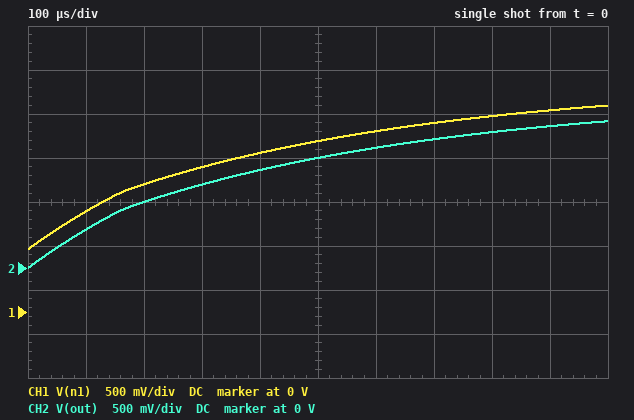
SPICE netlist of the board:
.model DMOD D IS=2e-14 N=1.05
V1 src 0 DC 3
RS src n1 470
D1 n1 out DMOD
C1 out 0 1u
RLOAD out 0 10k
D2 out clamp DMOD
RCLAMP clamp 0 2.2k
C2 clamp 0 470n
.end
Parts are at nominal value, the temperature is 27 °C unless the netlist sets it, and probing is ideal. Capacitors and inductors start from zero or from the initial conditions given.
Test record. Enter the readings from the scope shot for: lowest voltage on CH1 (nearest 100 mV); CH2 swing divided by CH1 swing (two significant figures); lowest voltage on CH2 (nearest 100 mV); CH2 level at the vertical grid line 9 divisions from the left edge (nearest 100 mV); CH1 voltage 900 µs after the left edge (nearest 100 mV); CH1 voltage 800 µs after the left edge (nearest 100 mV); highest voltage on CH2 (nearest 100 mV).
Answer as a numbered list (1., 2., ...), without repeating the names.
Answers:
1. 700 mV
2. 1.0
3. 0 V
4. 1.6 V
5. 2.3 V
6. 2.2 V
7. 1.7 V
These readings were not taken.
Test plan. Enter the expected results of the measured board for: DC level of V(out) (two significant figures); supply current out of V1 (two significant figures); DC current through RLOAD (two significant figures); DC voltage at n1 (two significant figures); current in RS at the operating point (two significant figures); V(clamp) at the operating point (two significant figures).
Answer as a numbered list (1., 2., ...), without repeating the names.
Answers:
1. 2.0 V
2. 790 µA
3. 200 µA
4. 2.6 V
5. 790 µA
6. 1.3 V
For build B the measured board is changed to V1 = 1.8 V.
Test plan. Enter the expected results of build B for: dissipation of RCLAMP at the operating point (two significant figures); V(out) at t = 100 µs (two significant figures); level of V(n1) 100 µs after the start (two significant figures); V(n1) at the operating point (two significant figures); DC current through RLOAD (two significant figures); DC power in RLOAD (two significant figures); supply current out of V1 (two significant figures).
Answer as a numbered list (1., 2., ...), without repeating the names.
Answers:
1. 75 µW
2. 210 mV
3. 900 mV
4. 1.7 V
5. 100 µA
6. 110 µW
7. 290 µA
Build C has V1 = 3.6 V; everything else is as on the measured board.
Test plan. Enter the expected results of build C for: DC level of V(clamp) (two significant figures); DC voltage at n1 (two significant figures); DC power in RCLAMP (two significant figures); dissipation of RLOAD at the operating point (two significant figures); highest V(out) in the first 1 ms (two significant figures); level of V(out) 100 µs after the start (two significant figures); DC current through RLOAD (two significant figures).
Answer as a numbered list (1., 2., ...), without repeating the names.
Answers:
1. 1.8 V
2. 3.1 V
3. 1.4 mW
4. 590 µW
5. 2.1 V
6. 550 mV
7. 240 µA
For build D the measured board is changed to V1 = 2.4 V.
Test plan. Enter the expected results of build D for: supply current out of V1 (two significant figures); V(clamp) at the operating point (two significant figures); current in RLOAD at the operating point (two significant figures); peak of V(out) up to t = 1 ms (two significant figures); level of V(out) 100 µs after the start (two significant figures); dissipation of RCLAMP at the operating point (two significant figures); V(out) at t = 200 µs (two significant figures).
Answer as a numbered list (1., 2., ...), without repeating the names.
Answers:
1. 540 µA
2. 850 mV
3. 150 µA
4. 1.3 V
5. 320 mV
6. 330 µW
7. 580 mV
